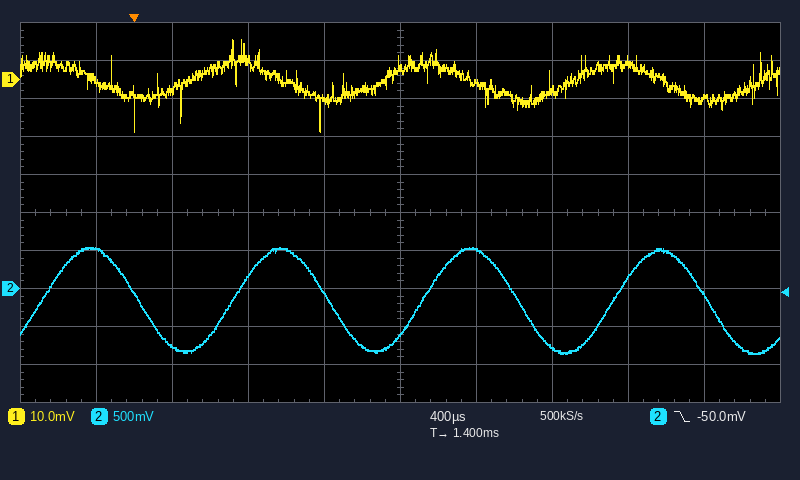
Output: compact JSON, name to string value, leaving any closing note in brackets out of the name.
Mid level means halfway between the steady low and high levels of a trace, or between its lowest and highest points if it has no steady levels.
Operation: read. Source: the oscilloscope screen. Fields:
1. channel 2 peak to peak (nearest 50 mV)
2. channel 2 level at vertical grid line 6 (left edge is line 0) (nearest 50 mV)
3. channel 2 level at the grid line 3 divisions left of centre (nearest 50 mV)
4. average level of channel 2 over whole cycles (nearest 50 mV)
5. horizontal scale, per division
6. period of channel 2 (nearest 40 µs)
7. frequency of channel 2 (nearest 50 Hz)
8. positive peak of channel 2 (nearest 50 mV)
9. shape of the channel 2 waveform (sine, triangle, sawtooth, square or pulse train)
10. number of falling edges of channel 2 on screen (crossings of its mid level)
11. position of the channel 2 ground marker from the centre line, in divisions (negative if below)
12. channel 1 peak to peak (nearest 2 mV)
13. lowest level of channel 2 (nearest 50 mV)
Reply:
{"channel 2 peak to peak": "1.40 V", "channel 2 level at vertical grid line 6 (left edge is line 0)": "500 mV", "channel 2 level at the grid line 3 divisions left of centre": "-750 mV", "average level of channel 2 over whole cycles": "-150 mV", "horizontal scale, per division": "400 µs", "period of channel 2": "1.00 ms", "frequency of channel 2": "1.00 kHz", "positive peak of channel 2": "550 mV", "shape of the channel 2 waveform": "sine", "number of falling edges of channel 2 on screen": "4", "position of the channel 2 ground marker from the centre line, in divisions": "-2.0 div", "channel 1 peak to peak": "24 mV", "lowest level of channel 2": "-850 mV"}
